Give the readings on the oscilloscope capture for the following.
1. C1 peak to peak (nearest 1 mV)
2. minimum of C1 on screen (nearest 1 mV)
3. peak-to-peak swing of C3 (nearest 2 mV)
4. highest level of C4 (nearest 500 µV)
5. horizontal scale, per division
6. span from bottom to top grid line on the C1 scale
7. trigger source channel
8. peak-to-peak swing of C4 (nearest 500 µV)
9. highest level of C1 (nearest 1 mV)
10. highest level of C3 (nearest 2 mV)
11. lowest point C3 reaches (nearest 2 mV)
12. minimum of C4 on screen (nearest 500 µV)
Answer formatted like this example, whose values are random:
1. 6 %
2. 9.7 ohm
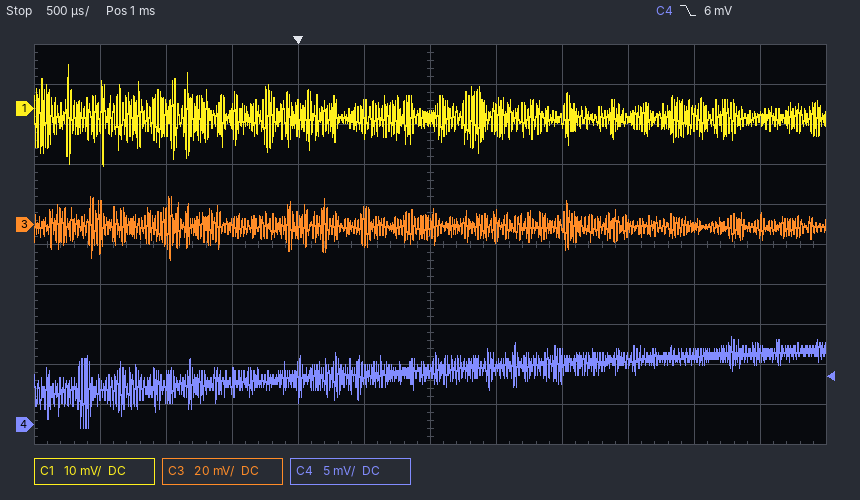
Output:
1. 25 mV
2. -14 mV
3. 32 mV
4. 11.0 mV
5. 500 µs
6. 100 mV
7. C4
8. 11.5 mV
9. 11 mV
10. 14 mV
11. -18 mV
12. -500 µV
